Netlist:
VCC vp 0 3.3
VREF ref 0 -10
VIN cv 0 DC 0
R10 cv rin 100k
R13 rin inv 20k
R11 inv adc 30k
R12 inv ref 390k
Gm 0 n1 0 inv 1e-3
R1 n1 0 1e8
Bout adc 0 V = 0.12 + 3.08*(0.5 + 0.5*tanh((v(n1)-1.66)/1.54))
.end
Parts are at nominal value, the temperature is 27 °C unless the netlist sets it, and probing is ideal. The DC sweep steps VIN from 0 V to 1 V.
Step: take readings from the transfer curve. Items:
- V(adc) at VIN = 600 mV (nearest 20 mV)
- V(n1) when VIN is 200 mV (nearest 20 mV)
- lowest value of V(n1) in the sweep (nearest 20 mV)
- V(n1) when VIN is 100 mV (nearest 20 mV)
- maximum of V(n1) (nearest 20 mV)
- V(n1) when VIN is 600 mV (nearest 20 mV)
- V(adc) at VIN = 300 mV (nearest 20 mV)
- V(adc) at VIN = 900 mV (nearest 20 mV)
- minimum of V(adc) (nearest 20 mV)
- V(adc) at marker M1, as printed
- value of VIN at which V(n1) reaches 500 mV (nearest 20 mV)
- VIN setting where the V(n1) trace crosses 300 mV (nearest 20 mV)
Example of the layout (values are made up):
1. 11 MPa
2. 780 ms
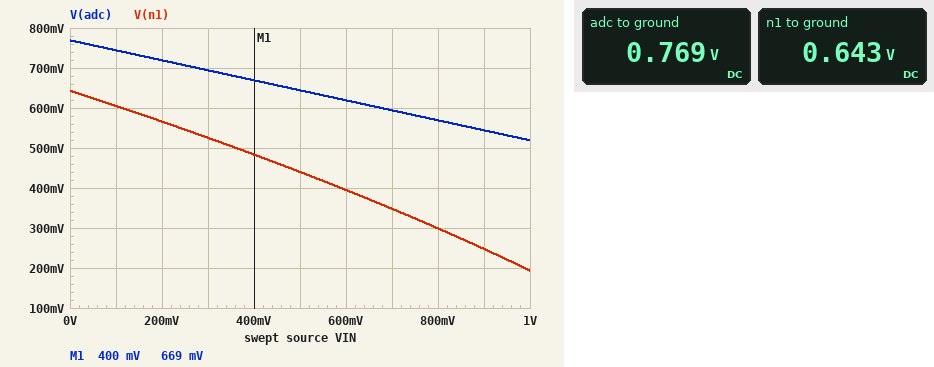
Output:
1. 620 mV
2. 560 mV
3. 200 mV
4. 600 mV
5. 640 mV
6. 400 mV
7. 700 mV
8. 540 mV
9. 520 mV
10. 669 mV
11. 360 mV
12. 800 mV
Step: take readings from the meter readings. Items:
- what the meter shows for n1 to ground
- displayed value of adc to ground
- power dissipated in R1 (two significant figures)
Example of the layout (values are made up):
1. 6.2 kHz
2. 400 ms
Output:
1. 0.643 V
2. 0.769 V
3. 4.1 nW
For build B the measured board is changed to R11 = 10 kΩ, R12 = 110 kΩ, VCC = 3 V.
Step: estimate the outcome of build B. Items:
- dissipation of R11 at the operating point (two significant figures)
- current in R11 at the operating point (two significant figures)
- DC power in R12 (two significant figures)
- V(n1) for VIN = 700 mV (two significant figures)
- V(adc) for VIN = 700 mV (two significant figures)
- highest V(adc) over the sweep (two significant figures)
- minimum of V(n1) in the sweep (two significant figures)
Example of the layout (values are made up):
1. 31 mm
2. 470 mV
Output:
1. 83 µW
2. 91 µA
3. 910 µW
4. 760 mV
5. 850 mV
6. 910 mV
7. 730 mV
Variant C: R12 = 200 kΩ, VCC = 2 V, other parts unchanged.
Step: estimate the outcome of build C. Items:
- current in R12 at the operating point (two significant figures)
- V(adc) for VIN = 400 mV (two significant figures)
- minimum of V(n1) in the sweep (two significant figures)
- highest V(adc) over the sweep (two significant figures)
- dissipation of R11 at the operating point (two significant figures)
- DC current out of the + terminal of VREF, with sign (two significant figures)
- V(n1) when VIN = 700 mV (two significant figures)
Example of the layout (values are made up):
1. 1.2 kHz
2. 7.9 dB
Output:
1. 50 µA
2. 1.4 V
3. 1.2 V
4. 1.5 V
5. 75 µW
6. -50 µA
7. 1.3 V
